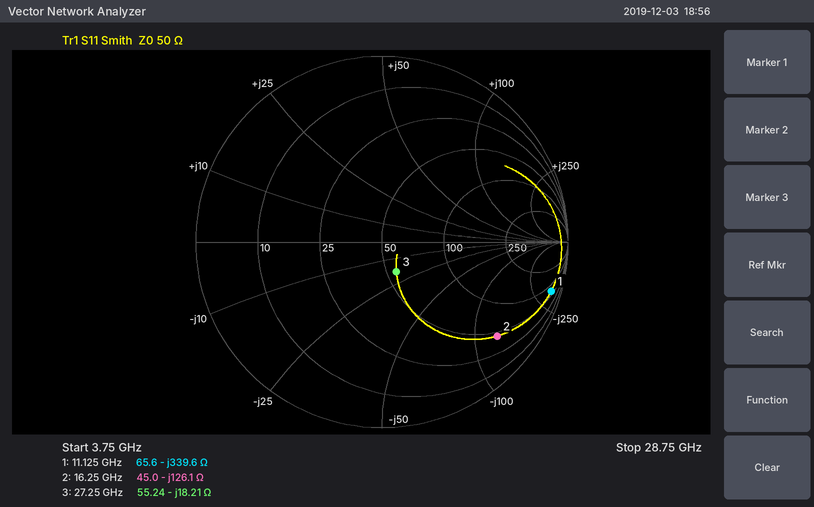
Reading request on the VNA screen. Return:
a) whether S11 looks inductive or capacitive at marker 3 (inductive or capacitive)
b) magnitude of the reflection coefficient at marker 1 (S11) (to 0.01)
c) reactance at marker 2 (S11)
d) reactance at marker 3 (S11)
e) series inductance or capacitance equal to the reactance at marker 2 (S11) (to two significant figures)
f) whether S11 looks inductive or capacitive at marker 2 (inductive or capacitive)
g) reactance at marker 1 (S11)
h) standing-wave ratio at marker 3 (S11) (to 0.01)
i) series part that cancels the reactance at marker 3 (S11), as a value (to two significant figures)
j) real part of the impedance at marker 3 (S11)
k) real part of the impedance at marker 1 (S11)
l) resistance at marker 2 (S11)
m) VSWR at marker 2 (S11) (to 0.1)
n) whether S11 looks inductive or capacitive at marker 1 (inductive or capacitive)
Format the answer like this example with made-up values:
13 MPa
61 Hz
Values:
capacitive
0.95
-126.1 Ω
-18.21 Ω
78 fF
capacitive
-339.6 Ω
1.43
110 pH
55.24 Ω
65.6 Ω
45.0 Ω
9.0
capacitive
